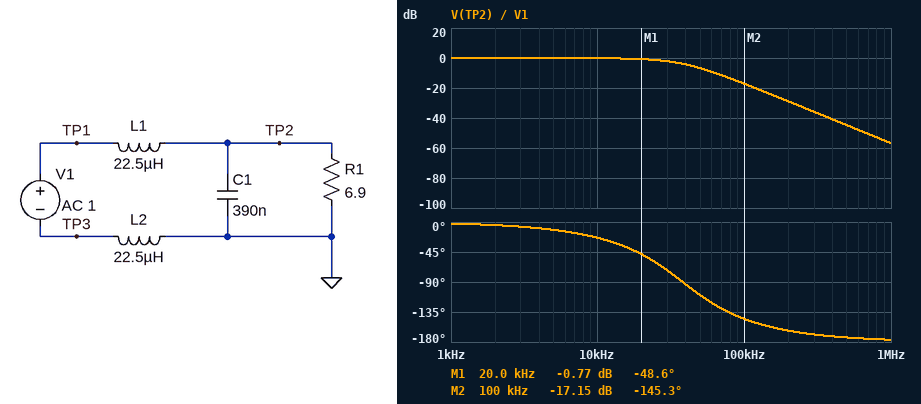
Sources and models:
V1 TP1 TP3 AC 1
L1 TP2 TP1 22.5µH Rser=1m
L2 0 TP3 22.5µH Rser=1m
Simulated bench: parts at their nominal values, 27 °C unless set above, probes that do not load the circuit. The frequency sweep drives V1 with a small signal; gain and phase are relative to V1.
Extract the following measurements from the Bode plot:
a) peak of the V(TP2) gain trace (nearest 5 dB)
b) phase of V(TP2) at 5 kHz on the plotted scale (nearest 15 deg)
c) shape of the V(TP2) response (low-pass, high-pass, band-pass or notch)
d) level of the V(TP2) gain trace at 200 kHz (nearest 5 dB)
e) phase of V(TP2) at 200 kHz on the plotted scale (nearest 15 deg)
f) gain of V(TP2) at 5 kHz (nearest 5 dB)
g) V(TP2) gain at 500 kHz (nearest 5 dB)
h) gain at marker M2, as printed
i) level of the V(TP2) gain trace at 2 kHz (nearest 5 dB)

0 dB
-15 deg
low-pass
-30 dB
-165 deg
0 dB
-45 dB
-17.15 dB
0 dB
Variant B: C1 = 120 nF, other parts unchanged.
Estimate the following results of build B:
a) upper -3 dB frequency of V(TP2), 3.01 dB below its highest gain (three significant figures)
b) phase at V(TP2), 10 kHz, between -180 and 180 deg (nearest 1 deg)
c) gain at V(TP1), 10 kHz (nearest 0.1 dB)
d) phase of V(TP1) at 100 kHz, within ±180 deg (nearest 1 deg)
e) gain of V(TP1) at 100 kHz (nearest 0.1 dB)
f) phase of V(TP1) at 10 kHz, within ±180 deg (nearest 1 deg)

27.9 kHz
-23 deg
-0.4 dB
-14 deg
-6.3 dB
-11 deg
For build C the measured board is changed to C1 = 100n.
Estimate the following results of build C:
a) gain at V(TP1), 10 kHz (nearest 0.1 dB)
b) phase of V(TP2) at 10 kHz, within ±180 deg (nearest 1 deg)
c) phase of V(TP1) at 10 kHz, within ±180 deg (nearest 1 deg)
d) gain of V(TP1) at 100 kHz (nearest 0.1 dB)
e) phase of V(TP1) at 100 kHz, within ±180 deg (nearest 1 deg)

-0.4 dB
-23 deg
-11 deg
-6.2 dB
-14 deg
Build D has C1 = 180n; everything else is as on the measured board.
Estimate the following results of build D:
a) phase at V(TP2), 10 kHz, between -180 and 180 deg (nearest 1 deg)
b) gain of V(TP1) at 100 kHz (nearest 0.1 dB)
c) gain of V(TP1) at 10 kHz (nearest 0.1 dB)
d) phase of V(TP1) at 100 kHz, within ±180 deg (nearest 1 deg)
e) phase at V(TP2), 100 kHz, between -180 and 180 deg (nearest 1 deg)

-23 deg
-6.8 dB
-0.4 dB
-12 deg
-118 deg
